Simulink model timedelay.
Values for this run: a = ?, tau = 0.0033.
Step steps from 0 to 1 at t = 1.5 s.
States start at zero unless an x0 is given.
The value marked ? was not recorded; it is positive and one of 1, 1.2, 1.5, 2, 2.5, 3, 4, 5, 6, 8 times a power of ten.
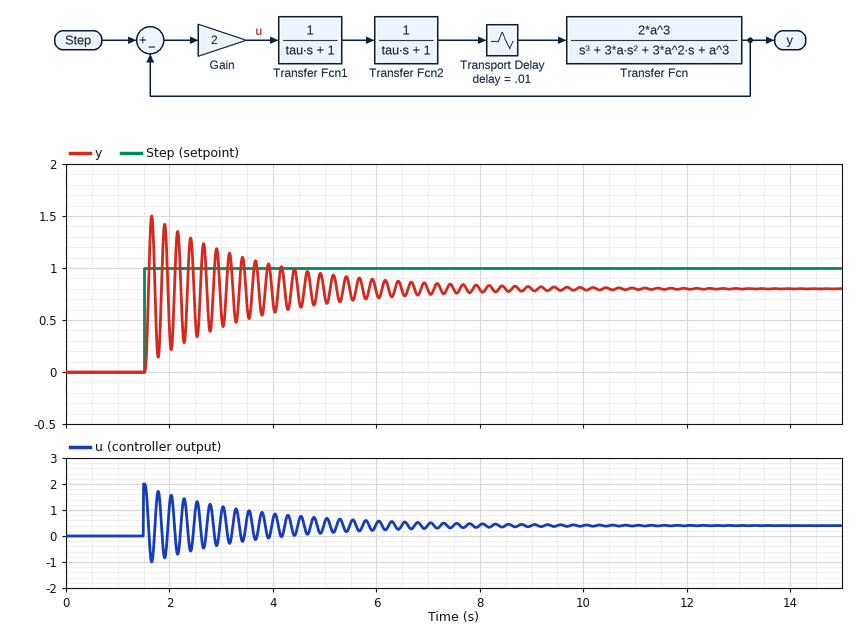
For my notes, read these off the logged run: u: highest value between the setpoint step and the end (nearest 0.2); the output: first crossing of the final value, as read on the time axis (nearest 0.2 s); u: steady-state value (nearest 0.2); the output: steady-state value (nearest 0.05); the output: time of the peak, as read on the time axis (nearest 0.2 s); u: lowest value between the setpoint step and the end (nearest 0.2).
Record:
2.0
1.6 s
0.4
0.80
1.6 s
-1.0
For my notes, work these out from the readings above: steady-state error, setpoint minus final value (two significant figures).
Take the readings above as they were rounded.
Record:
0.20
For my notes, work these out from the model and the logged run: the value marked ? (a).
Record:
20
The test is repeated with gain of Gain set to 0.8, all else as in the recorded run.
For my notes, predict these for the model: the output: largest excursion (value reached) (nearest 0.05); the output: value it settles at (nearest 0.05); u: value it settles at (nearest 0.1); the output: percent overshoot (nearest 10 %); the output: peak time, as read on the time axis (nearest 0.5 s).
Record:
0.85
0.60
0.3
40 %
1.5 s
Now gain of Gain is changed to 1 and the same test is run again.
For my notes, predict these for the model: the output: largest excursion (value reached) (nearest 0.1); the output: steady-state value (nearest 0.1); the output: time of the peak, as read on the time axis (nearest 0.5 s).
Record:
1.0
0.7
1.5 s
